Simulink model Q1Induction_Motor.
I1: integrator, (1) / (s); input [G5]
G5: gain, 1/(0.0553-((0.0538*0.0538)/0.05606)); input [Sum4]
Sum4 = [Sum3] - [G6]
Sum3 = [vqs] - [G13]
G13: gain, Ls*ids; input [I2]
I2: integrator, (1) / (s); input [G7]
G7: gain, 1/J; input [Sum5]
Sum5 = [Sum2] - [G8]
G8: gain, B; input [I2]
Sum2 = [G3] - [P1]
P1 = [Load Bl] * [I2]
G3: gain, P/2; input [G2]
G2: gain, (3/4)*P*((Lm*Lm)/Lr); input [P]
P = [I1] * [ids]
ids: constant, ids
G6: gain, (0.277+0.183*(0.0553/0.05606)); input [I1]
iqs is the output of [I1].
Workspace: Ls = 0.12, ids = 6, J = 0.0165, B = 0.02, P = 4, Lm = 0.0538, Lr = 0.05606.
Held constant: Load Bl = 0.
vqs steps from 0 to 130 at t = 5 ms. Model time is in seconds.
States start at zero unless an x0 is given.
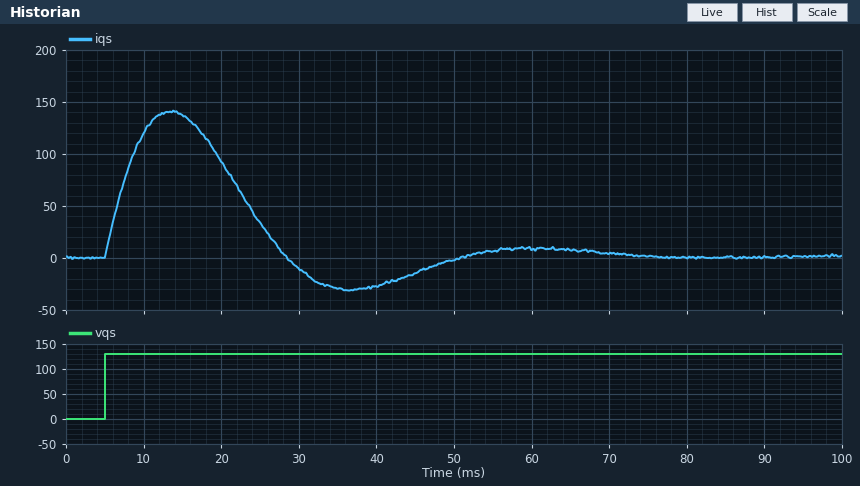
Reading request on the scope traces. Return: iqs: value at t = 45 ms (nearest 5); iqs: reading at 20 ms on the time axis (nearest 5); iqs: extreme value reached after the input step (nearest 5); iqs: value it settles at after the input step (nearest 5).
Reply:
-15
95
140
0
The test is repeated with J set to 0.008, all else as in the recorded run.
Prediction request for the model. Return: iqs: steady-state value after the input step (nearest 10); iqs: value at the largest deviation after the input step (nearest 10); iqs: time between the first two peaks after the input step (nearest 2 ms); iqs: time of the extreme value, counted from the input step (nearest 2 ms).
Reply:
0
110
30 ms
6 ms
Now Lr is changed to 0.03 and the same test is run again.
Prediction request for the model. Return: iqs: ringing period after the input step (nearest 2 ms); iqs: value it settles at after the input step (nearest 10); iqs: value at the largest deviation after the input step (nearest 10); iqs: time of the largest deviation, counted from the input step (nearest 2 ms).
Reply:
32 ms
0
120
6 ms
